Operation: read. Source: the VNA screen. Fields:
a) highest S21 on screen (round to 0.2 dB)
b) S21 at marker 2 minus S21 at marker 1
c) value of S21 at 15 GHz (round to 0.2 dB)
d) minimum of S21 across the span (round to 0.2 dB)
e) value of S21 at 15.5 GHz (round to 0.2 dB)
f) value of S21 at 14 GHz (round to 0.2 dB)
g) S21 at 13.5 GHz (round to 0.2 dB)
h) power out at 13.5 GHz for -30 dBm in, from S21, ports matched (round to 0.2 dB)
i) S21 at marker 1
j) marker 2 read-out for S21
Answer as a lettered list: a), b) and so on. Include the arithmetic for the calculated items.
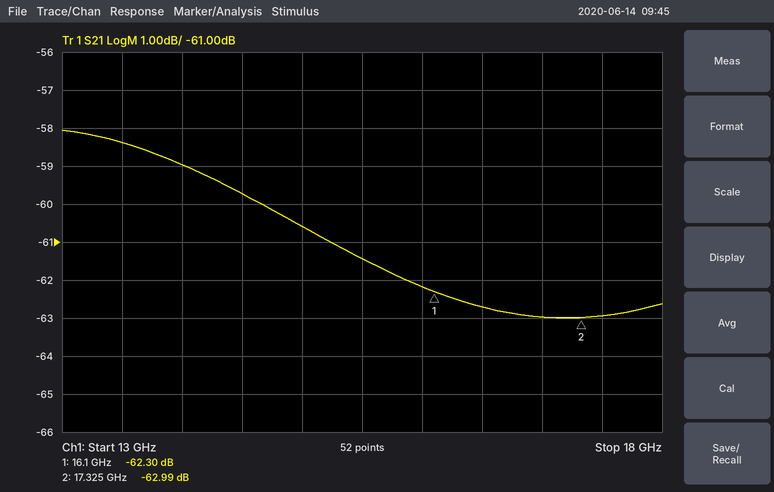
a) -58.0 dB
b) -62.99 − (-62.3) = -0.69 dB
c) -60.6 dB
d) -63.0 dB
e) -61.4 dB
f) -59.0 dB
g) -58.4 dB
h) -30 dBm + (-58.4 dB) = -88.4 dBm
i) -62.30 dB
j) -62.99 dB
